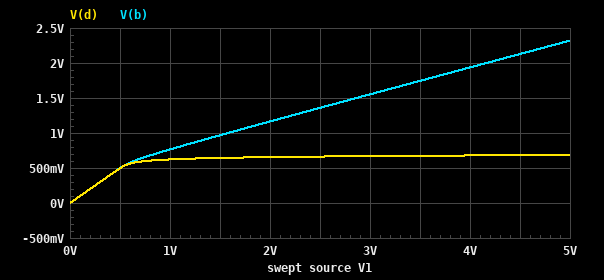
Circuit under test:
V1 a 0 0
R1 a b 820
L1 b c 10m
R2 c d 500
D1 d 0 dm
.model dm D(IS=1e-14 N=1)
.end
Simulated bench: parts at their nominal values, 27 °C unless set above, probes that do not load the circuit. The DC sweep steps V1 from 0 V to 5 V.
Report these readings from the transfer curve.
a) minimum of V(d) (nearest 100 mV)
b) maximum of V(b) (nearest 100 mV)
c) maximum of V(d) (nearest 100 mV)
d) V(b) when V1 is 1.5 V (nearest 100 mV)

0 V
2.3 V
700 mV
1.0 V
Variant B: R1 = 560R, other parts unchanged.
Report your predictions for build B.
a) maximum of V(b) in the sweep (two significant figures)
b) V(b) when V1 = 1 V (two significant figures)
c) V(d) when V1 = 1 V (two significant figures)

2.7 V
800 mV
630 mV
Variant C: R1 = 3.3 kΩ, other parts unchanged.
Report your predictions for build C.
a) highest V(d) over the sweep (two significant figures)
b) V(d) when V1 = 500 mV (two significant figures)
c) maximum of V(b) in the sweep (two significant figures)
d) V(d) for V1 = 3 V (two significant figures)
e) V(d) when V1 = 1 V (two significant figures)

660 mV
490 mV
1.2 V
640 mV
600 mV
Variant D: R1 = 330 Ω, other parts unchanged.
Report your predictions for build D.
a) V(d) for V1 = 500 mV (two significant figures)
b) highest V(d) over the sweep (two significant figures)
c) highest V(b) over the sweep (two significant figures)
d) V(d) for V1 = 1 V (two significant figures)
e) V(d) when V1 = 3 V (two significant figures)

500 mV
700 mV
3.3 V
630 mV
680 mV
